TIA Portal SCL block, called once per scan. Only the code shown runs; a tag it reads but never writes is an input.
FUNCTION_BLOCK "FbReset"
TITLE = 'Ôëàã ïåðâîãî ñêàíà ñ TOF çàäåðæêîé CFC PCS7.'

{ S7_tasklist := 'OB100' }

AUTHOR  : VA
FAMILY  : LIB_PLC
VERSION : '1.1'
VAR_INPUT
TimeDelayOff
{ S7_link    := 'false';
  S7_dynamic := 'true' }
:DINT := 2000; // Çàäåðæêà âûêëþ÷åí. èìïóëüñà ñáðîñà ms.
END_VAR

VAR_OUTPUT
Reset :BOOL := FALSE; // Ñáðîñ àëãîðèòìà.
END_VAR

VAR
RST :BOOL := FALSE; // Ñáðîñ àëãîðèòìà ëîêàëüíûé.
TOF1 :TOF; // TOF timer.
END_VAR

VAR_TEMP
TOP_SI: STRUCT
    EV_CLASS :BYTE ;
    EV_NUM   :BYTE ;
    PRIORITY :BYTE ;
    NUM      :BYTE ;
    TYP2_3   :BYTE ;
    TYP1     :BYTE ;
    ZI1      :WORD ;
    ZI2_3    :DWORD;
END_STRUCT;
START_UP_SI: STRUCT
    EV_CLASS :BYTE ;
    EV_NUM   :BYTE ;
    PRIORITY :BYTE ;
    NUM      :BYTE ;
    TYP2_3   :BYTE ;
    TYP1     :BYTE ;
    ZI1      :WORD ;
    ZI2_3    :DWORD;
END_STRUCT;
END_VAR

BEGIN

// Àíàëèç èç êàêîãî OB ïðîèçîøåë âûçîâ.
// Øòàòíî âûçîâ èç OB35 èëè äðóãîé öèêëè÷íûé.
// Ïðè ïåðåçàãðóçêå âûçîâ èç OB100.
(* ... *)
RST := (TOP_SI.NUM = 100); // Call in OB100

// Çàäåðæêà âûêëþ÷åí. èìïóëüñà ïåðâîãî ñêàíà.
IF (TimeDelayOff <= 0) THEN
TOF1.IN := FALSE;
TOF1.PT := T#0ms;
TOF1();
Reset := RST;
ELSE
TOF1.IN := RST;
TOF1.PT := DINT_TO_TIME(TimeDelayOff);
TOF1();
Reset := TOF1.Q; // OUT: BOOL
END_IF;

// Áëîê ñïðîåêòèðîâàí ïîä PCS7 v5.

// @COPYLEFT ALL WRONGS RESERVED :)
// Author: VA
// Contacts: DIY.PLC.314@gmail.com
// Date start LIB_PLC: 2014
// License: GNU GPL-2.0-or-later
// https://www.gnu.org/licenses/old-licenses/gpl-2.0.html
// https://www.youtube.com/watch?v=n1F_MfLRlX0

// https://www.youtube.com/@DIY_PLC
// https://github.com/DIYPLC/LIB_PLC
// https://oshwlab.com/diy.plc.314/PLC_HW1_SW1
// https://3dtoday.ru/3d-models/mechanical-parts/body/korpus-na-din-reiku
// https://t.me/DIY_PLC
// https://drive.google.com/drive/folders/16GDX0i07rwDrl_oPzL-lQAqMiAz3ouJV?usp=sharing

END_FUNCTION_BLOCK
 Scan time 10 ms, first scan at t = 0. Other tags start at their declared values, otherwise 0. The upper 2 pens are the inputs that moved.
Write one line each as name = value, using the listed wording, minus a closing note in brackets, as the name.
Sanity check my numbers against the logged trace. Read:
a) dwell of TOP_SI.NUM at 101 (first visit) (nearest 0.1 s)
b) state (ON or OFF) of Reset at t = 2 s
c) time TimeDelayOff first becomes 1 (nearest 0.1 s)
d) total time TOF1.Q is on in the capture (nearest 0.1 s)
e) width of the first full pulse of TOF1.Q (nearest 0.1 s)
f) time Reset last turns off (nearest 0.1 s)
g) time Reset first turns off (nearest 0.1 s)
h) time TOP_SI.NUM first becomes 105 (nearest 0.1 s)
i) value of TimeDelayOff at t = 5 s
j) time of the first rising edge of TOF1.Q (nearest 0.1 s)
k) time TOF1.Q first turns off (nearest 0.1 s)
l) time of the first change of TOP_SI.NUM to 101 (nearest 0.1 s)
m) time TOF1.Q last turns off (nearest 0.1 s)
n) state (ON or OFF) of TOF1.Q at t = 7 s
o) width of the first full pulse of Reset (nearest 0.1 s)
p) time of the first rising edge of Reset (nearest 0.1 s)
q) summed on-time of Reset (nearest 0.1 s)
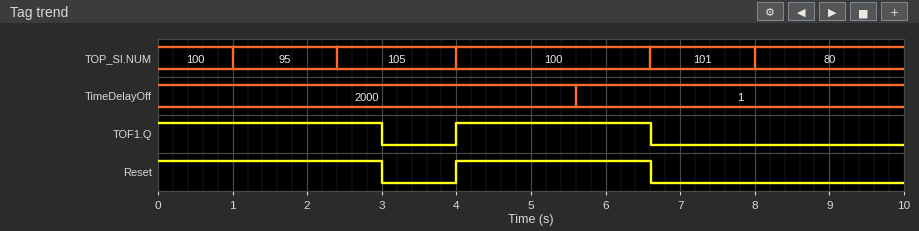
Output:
dwell of TOP_SI.NUM at 101 (first visit) = 1.4 s
state (ON or OFF) of Reset at t = 2 s = ON
time TimeDelayOff first becomes 1 = 5.6 s
total time TOF1.Q is on in the capture = 5.6 s
width of the first full pulse of TOF1.Q = 2.6 s
time Reset last turns off = 6.6 s
time Reset first turns off = 3.0 s
time TOP_SI.NUM first becomes 105 = 2.4 s
value of TimeDelayOff at t = 5 s = 2000
time of the first rising edge of TOF1.Q = 4.0 s
time TOF1.Q first turns off = 3.0 s
time of the first change of TOP_SI.NUM to 101 = 6.6 s
time TOF1.Q last turns off = 6.6 s
state (ON or OFF) of TOF1.Q at t = 7 s = OFF
width of the first full pulse of Reset = 2.6 s
time of the first rising edge of Reset = 4.0 s
summed on-time of Reset = 5.6 s
